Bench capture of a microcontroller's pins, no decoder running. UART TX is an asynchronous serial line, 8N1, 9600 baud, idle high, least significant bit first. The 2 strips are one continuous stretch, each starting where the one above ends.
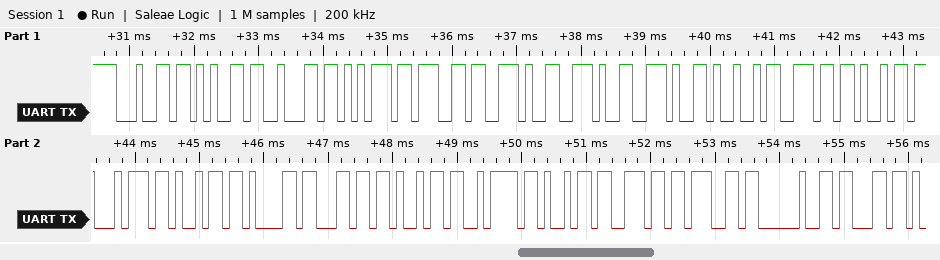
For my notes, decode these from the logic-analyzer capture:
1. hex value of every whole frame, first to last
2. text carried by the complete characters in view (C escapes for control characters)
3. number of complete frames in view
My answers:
64 65 62 75 67 2E 2E 2E 49 6E 69 74 69 61 6C 69 7A 69 6E 67 20 63
"debug...Initializing c"
22
